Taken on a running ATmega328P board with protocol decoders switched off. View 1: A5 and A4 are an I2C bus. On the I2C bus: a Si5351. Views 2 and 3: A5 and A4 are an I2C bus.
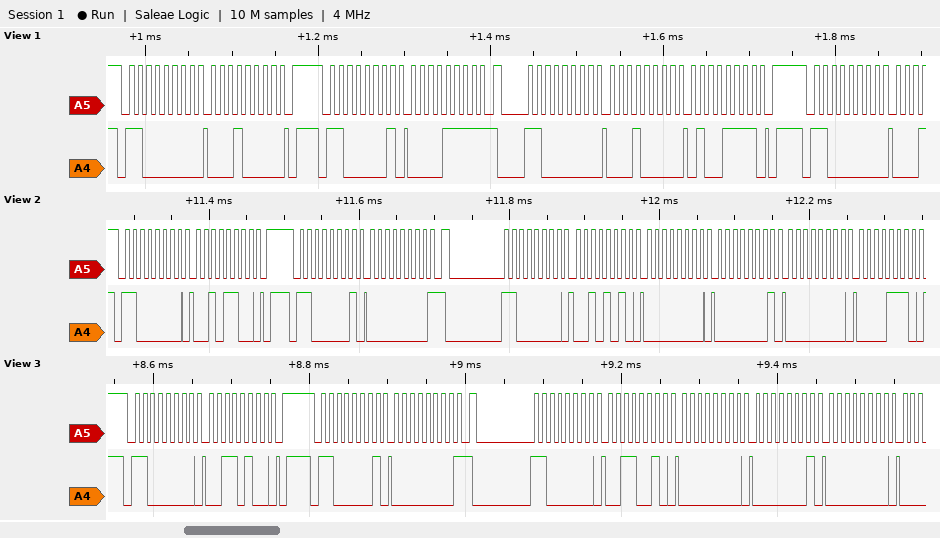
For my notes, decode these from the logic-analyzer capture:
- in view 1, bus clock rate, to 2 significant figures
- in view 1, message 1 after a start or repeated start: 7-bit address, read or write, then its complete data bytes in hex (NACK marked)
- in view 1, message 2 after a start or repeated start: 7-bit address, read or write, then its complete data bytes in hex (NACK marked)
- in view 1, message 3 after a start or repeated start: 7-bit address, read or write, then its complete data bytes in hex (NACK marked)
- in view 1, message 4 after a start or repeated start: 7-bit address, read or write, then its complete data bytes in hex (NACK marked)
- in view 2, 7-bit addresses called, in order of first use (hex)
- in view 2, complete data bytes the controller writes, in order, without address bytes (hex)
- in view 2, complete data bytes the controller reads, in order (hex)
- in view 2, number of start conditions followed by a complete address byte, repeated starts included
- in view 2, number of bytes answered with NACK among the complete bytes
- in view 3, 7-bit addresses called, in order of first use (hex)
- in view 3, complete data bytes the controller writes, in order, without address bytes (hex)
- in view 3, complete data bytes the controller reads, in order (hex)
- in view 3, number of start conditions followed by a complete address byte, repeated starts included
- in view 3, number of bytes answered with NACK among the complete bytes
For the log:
100 kHz
0x60 write: 10
0x60 read: 0F NACK
0x60 write: 10 4F
0x60 write
0x60
2C 2A 00 01 00 0E
00
3
1
0x60
34 32 00 01 00
00
3
1
